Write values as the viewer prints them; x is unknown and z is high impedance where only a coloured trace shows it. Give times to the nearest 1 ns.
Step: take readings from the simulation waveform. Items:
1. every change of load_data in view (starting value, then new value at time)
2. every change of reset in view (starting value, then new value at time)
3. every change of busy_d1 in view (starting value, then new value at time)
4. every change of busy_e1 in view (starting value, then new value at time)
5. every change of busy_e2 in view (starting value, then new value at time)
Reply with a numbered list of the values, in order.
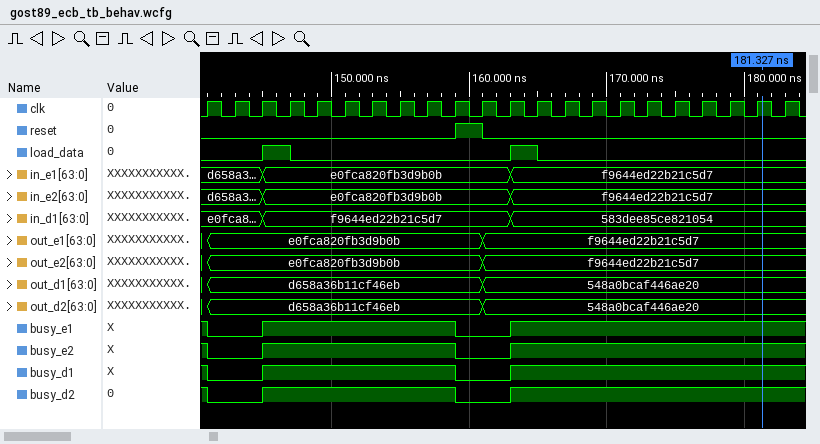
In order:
1. 0, 1 at 145 ns, 0 at 147 ns, 1 at 163 ns, 0 at 165 ns
2. 0, 1 at 159 ns, 0 at 161 ns
3. 1, 0 at 141 ns, 1 at 145 ns, 0 at 159 ns, 1 at 163 ns
4. 1, 0 at 141 ns, 1 at 145 ns, 0 at 159 ns, 1 at 163 ns
5. 1, 0 at 141 ns, 1 at 145 ns, 0 at 159 ns, 1 at 163 ns
